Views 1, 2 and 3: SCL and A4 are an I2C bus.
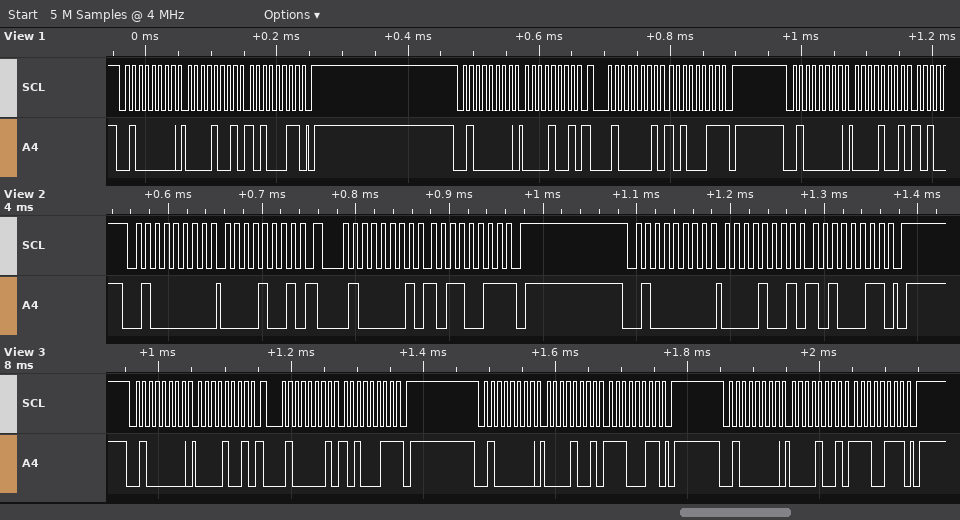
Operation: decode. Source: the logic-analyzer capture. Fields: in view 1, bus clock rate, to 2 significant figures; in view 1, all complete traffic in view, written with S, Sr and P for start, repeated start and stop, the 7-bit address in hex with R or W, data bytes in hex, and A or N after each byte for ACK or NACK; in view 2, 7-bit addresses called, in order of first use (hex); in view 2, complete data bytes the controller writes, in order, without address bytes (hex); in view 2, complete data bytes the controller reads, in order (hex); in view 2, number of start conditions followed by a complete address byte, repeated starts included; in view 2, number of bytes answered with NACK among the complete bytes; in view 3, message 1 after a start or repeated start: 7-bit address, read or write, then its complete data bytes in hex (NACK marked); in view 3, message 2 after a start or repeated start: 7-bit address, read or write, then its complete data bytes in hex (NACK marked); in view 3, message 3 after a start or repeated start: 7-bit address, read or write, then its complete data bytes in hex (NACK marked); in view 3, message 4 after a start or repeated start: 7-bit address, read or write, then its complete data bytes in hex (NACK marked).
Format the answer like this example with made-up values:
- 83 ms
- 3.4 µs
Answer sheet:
- 100 kHz
- S 20W A 09 A A3 A P S 20W A 09 A Sr 20R A A3 N P S 20W A 09 A
- 0x20
- 09 09 A3
- B3
- 3
- 1
- 0x20 write: 09
- 0x20 read: A3 NACK
- 0x20 write: 09 E3
- 0x20 write: 09 E7
